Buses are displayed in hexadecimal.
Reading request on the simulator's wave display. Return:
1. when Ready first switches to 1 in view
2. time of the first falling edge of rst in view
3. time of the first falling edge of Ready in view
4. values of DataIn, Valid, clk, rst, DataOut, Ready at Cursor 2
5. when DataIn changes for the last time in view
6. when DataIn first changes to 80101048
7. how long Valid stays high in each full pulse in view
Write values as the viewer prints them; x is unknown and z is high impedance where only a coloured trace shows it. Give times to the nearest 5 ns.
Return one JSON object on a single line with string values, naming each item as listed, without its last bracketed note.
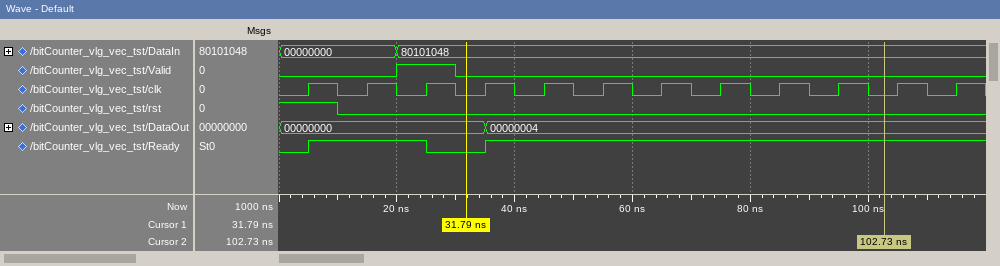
{"when Ready first switches to 1 in view": "5 ns", "time of the first falling edge of rst in view": "10 ns", "time of the first falling edge of Ready in view": "25 ns", "values of DataIn, Valid, clk, rst, DataOut, Ready at Cursor 2": "DataIn=80101048, Valid=0, clk=0, rst=0, DataOut=00000004, Ready=1", "when DataIn changes for the last time in view": "20 ns", "when DataIn first changes to 80101048": "20 ns", "how long Valid stays high in each full pulse in view": "10 ns"}
